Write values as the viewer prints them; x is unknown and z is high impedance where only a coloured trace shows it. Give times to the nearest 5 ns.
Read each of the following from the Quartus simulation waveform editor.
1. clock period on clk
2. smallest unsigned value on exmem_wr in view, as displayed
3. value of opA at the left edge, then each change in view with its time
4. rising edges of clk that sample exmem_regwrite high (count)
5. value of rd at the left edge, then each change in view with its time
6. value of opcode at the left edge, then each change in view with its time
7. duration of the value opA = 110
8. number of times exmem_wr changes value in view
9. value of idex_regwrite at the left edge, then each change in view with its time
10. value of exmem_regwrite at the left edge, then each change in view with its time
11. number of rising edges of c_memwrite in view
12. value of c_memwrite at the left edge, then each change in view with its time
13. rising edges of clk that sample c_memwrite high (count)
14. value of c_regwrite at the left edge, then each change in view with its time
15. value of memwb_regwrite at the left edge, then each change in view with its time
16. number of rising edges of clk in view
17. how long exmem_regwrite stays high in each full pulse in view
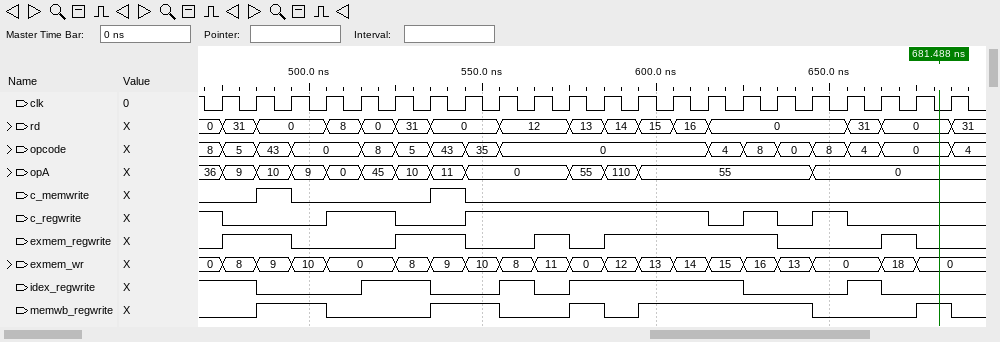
10 ns
0
36, 9 at 475 ns, 10 at 485 ns, 9 at 495 ns, 0 at 505 ns, 45 at 515 ns, 10 at 525 ns, 11 at 535 ns, 0 at 545 ns, 55 at 575 ns, 110 at 585 ns, 55 at 595 ns, 0 at 645 ns
11
0, 31 at 475 ns, 0 at 485 ns, 8 at 505 ns, 0 at 515 ns, 31 at 525 ns, 0 at 535 ns, 12 at 555 ns, 13 at 575 ns, 14 at 585 ns, 15 at 595 ns, 16 at 605 ns, 0 at 615 ns, 31 at 655 ns, 0 at 665 ns, 31 at 685 ns
8, 5 at 475 ns, 43 at 485 ns, 0 at 495 ns, 8 at 515 ns, 5 at 525 ns, 43 at 535 ns, 35 at 545 ns, 0 at 555 ns, 4 at 615 ns, 8 at 625 ns, 0 at 635 ns, 8 at 645 ns, 4 at 655 ns, 0 at 665 ns, 4 at 685 ns
10 ns
19
1, 0 at 485 ns, 1 at 515 ns, 0 at 535 ns, 1 at 555 ns, 0 at 565 ns, 1 at 575 ns, 0 at 625 ns, 1 at 655 ns, 0 at 665 ns
0, 1 at 475 ns, 0 at 495 ns, 1 at 525 ns, 0 at 545 ns, 1 at 565 ns, 0 at 575 ns, 1 at 585 ns, 0 at 635 ns, 1 at 665 ns, 0 at 675 ns
2
0, 1 at 485 ns, 0 at 495 ns, 1 at 535 ns, 0 at 545 ns
2
1, 0 at 475 ns, 1 at 505 ns, 0 at 525 ns, 1 at 545 ns, 0 at 615 ns, 1 at 625 ns, 0 at 635 ns, 1 at 645 ns, 0 at 655 ns
0, 1 at 485 ns, 0 at 505 ns, 1 at 535 ns, 0 at 555 ns, 1 at 575 ns, 0 at 585 ns, 1 at 595 ns, 0 at 645 ns, 1 at 675 ns, 0 at 685 ns
22
20 ns, 20 ns, 10 ns, 50 ns, 10 ns
